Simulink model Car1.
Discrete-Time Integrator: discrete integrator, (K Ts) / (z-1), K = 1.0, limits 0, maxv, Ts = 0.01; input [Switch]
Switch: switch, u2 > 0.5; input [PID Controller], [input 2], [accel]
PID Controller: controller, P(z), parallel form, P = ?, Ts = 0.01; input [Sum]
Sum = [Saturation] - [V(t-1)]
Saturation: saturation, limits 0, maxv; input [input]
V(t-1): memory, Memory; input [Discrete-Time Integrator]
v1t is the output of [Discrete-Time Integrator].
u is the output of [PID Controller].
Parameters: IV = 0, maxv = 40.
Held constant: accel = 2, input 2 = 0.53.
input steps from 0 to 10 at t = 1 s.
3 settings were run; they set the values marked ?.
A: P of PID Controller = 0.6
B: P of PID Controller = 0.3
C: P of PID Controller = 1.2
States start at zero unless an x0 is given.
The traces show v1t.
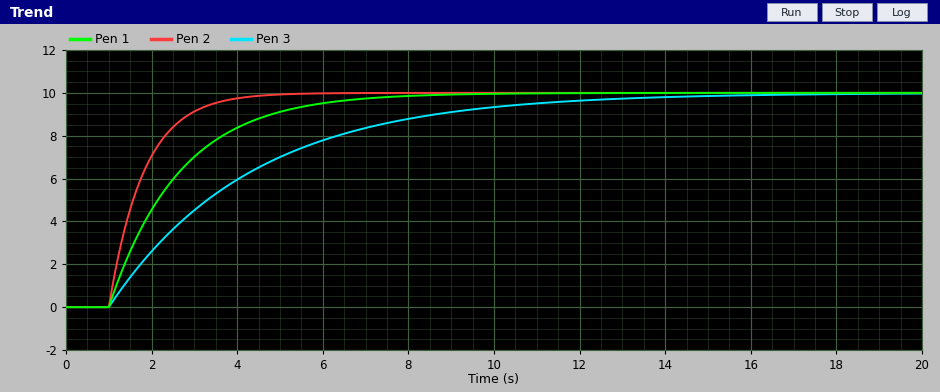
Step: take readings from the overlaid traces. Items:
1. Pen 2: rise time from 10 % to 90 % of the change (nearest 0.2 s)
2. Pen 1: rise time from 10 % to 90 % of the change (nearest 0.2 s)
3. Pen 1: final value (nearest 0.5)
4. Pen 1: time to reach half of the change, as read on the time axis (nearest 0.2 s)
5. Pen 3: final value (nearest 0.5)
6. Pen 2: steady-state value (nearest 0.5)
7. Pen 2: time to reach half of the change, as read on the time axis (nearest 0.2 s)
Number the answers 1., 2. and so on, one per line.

1. 1.8 s
2. 3.6 s
3. 10.0
4. 2.2 s
5. 10.0
6. 10.0
7. 1.6 s
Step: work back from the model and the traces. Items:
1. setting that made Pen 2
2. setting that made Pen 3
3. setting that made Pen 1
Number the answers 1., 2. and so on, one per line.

1. C
2. B
3. A
